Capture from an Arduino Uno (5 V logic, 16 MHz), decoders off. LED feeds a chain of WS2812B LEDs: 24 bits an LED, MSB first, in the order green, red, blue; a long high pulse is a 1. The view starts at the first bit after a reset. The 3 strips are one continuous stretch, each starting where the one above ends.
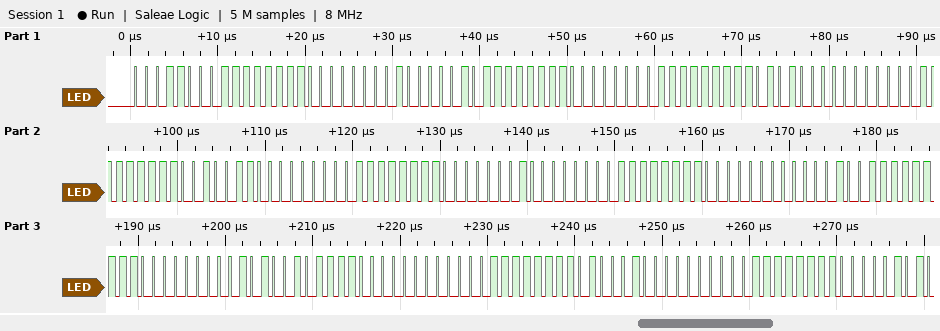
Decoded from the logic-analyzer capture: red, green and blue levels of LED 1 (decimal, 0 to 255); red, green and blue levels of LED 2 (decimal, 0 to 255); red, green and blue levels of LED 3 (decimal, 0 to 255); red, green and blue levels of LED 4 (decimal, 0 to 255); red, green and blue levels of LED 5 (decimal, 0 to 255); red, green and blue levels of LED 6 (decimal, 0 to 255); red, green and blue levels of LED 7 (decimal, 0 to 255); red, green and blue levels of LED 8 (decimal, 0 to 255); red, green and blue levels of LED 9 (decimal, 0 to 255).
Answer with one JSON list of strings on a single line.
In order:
["255, 24, 0", "255, 130, 0", "168, 255, 0", "38, 255, 0", "1, 255, 0", "0, 255, 9", "0, 255, 82", "0, 240, 255", "0, 68, 255"]
